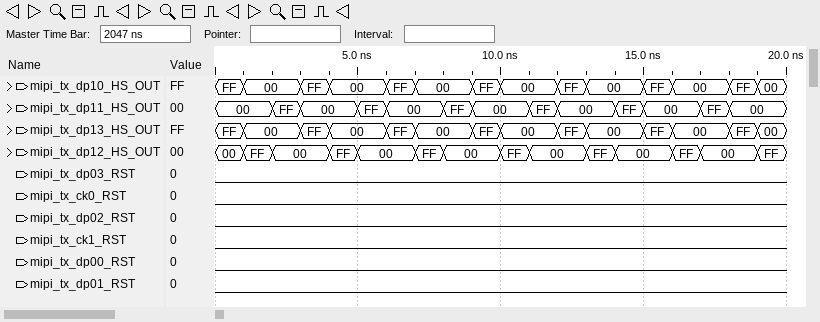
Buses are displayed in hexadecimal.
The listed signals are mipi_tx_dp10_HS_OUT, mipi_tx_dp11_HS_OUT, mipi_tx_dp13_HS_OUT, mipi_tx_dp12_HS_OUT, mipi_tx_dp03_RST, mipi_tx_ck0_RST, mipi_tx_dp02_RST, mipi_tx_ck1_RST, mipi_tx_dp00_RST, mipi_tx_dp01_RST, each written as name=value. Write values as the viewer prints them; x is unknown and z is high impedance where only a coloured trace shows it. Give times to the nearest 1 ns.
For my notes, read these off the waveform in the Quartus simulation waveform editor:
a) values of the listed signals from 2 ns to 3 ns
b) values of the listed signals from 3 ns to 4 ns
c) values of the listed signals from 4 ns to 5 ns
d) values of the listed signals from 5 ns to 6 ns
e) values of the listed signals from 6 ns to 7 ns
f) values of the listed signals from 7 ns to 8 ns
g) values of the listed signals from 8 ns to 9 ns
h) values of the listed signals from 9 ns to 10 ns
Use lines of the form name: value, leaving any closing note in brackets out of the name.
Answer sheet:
values of the listed signals from 2 ns to 3 ns: mipi_tx_dp10_HS_OUT=00, mipi_tx_dp11_HS_OUT=FF, mipi_tx_dp13_HS_OUT=00, mipi_tx_dp12_HS_OUT=00, mipi_tx_dp03_RST=0, mipi_tx_ck0_RST=0, mipi_tx_dp02_RST=0, mipi_tx_ck1_RST=0, mipi_tx_dp00_RST=0, mipi_tx_dp01_RST=0
values of the listed signals from 3 ns to 4 ns: mipi_tx_dp10_HS_OUT=FF, mipi_tx_dp11_HS_OUT=00, mipi_tx_dp13_HS_OUT=FF, mipi_tx_dp12_HS_OUT=00, mipi_tx_dp03_RST=0, mipi_tx_ck0_RST=0, mipi_tx_dp02_RST=0, mipi_tx_ck1_RST=0, mipi_tx_dp00_RST=0, mipi_tx_dp01_RST=0
values of the listed signals from 4 ns to 5 ns: mipi_tx_dp10_HS_OUT=00, mipi_tx_dp11_HS_OUT=00, mipi_tx_dp13_HS_OUT=00, mipi_tx_dp12_HS_OUT=FF, mipi_tx_dp03_RST=0, mipi_tx_ck0_RST=0, mipi_tx_dp02_RST=0, mipi_tx_ck1_RST=0, mipi_tx_dp00_RST=0, mipi_tx_dp01_RST=0
values of the listed signals from 5 ns to 6 ns: mipi_tx_dp10_HS_OUT=00, mipi_tx_dp11_HS_OUT=FF, mipi_tx_dp13_HS_OUT=00, mipi_tx_dp12_HS_OUT=00, mipi_tx_dp03_RST=0, mipi_tx_ck0_RST=0, mipi_tx_dp02_RST=0, mipi_tx_ck1_RST=0, mipi_tx_dp00_RST=0, mipi_tx_dp01_RST=0
values of the listed signals from 6 ns to 7 ns: mipi_tx_dp10_HS_OUT=FF, mipi_tx_dp11_HS_OUT=00, mipi_tx_dp13_HS_OUT=FF, mipi_tx_dp12_HS_OUT=00, mipi_tx_dp03_RST=0, mipi_tx_ck0_RST=0, mipi_tx_dp02_RST=0, mipi_tx_ck1_RST=0, mipi_tx_dp00_RST=0, mipi_tx_dp01_RST=0
values of the listed signals from 7 ns to 8 ns: mipi_tx_dp10_HS_OUT=00, mipi_tx_dp11_HS_OUT=00, mipi_tx_dp13_HS_OUT=00, mipi_tx_dp12_HS_OUT=FF, mipi_tx_dp03_RST=0, mipi_tx_ck0_RST=0, mipi_tx_dp02_RST=0, mipi_tx_ck1_RST=0, mipi_tx_dp00_RST=0, mipi_tx_dp01_RST=0
values of the listed signals from 8 ns to 9 ns: mipi_tx_dp10_HS_OUT=00, mipi_tx_dp11_HS_OUT=FF, mipi_tx_dp13_HS_OUT=00, mipi_tx_dp12_HS_OUT=00, mipi_tx_dp03_RST=0, mipi_tx_ck0_RST=0, mipi_tx_dp02_RST=0, mipi_tx_ck1_RST=0, mipi_tx_dp00_RST=0, mipi_tx_dp01_RST=0
values of the listed signals from 9 ns to 10 ns: mipi_tx_dp10_HS_OUT=FF, mipi_tx_dp11_HS_OUT=00, mipi_tx_dp13_HS_OUT=FF, mipi_tx_dp12_HS_OUT=00, mipi_tx_dp03_RST=0, mipi_tx_ck0_RST=0, mipi_tx_dp02_RST=0, mipi_tx_ck1_RST=0, mipi_tx_dp00_RST=0, mipi_tx_dp01_RST=0
